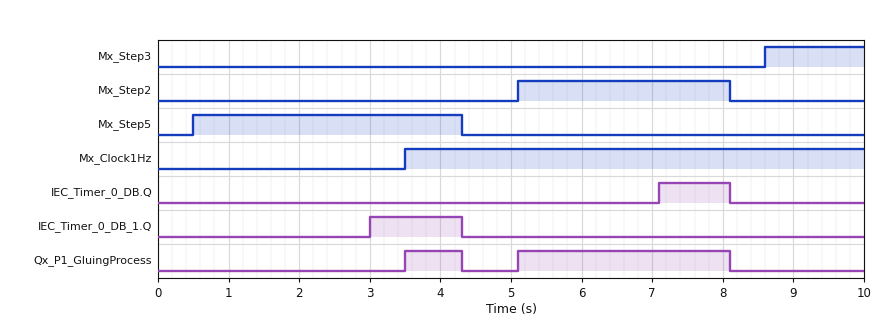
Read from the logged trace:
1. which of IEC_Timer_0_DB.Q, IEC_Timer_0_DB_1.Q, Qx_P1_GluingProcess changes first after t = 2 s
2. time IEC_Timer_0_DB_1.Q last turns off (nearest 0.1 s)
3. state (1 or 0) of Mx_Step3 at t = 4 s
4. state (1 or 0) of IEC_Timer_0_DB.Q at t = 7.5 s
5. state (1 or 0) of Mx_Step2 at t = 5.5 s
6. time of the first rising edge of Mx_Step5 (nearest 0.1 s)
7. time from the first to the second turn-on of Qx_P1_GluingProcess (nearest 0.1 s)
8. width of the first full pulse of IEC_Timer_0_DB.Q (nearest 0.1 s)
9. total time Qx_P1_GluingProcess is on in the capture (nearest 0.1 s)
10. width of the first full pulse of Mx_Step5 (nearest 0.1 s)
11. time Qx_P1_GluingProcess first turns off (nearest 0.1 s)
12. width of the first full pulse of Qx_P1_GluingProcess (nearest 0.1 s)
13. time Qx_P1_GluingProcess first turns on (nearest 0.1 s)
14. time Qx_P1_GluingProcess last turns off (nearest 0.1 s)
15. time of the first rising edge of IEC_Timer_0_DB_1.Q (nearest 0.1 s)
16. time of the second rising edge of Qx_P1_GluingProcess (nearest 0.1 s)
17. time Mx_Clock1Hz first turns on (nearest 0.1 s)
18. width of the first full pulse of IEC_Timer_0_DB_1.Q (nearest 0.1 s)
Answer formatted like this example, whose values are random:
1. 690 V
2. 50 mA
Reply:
1. IEC_Timer_0_DB_1.Q
2. 4.3 s
3. 0
4. 1
5. 1
6. 0.5 s
7. 1.6 s
8. 1.0 s
9. 3.8 s
10. 3.8 s
11. 4.3 s
12. 0.8 s
13. 3.5 s
14. 8.1 s
15. 3.0 s
16. 5.1 s
17. 3.5 s
18. 1.3 s
